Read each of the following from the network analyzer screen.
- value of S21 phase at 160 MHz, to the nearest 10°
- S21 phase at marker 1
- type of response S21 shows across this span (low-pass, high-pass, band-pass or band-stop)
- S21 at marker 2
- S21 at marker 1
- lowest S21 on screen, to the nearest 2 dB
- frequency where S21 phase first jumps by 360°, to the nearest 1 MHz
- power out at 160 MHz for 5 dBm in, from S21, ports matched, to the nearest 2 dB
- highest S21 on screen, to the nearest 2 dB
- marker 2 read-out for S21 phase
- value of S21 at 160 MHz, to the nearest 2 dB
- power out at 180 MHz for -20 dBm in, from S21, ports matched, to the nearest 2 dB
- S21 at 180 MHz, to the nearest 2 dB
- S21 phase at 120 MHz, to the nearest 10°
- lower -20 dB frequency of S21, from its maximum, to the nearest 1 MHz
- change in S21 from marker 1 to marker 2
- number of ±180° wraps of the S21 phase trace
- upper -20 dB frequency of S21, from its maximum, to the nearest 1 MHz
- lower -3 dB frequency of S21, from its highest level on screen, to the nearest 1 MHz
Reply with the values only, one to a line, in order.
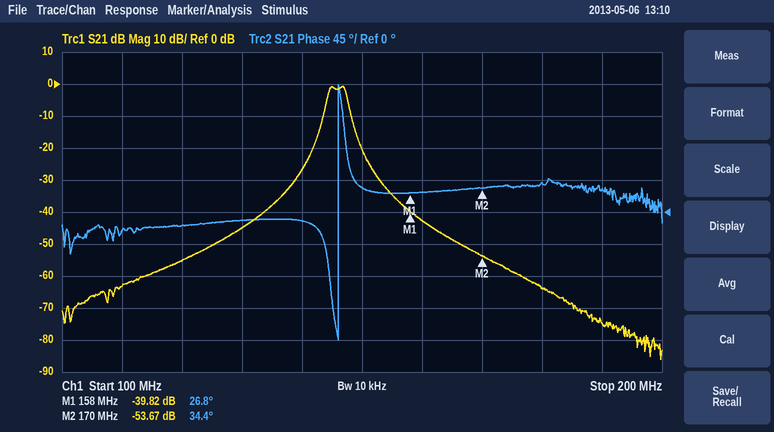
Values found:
30°
26.8°
band-pass
-53.67 dB
-39.82 dB
-86 dB
146 MHz
-38 dBm
0 dB
34.4°
-42 dB
-84 dBm
-64 dB
-20°
142 MHz
-13.85 dB
1
150 MHz
144 MHz
